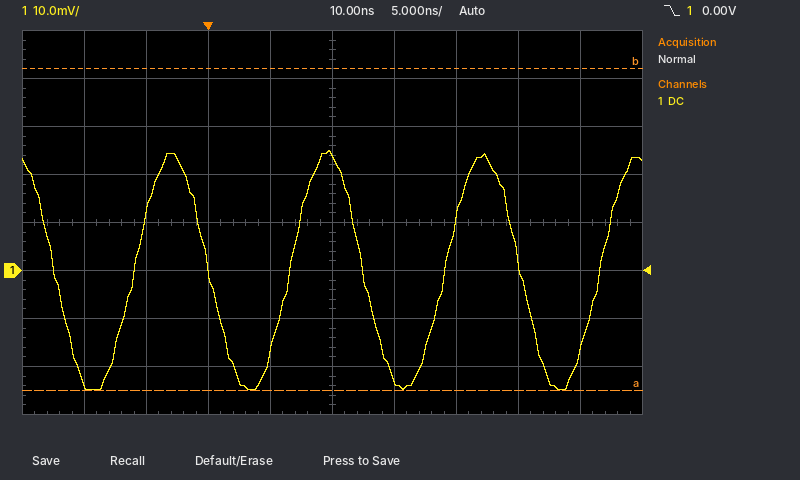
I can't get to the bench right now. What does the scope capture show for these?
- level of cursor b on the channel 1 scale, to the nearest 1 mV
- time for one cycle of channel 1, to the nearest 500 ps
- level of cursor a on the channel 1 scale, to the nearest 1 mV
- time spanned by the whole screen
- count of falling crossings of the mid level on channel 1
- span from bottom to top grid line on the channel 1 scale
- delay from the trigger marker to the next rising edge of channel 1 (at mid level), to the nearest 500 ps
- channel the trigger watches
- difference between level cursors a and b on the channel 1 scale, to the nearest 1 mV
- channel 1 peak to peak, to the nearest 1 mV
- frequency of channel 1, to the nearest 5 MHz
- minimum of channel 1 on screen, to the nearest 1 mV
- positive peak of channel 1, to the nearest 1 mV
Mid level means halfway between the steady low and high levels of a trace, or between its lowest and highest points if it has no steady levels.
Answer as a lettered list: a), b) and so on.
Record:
a) 42 mV
b) 12.5 ns
c) -25 mV
d) 50 ns
e) 4
f) 80 mV
g) 6.5 ns
h) channel 1
i) 67 mV
j) 50 mV
k) 80 MHz
l) -25 mV
m) 25 mV
